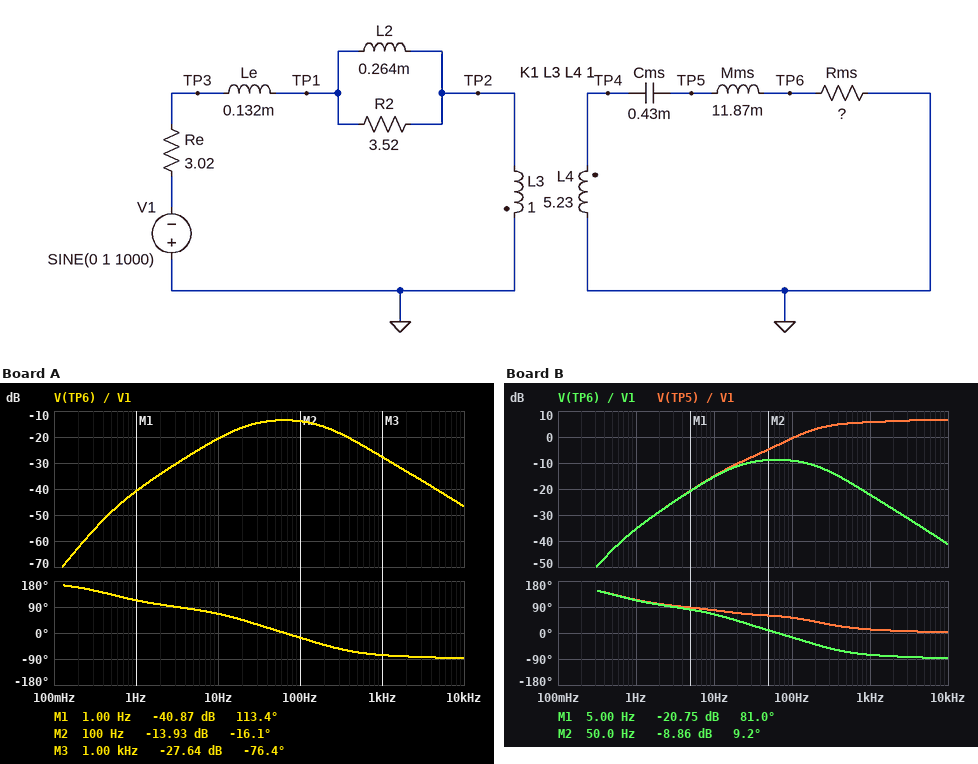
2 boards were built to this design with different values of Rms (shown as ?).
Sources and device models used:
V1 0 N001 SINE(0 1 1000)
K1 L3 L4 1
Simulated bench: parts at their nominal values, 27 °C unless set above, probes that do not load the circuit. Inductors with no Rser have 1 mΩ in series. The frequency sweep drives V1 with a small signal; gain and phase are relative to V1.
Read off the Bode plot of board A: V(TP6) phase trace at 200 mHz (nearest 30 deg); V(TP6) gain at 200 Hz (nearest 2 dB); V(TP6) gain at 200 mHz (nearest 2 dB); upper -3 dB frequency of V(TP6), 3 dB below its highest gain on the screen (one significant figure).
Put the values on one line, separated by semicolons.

150 deg; -16 dB; -62 dB; 200 Hz
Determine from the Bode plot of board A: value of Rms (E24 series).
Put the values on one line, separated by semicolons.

1.6 Ω
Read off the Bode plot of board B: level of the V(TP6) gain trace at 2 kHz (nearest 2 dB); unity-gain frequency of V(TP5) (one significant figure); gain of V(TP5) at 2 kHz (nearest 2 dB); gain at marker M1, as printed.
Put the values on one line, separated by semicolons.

-28 dB; 100 Hz; 6 dB; -20.75 dB
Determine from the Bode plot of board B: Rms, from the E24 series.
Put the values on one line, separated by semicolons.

3 Ω
